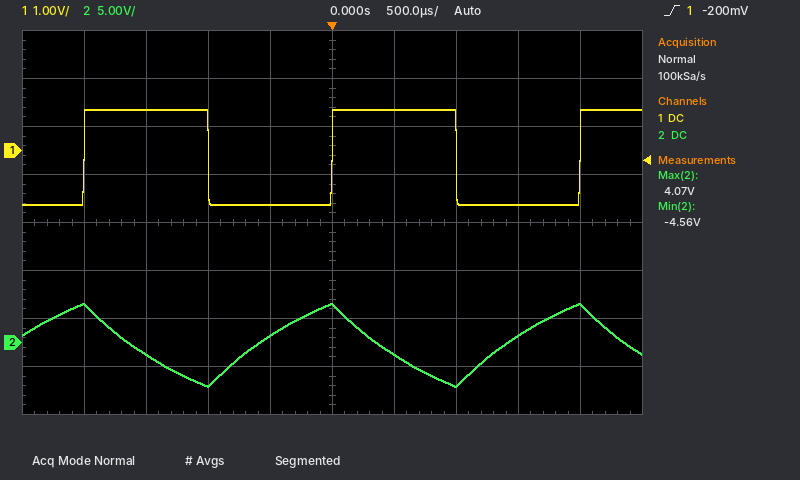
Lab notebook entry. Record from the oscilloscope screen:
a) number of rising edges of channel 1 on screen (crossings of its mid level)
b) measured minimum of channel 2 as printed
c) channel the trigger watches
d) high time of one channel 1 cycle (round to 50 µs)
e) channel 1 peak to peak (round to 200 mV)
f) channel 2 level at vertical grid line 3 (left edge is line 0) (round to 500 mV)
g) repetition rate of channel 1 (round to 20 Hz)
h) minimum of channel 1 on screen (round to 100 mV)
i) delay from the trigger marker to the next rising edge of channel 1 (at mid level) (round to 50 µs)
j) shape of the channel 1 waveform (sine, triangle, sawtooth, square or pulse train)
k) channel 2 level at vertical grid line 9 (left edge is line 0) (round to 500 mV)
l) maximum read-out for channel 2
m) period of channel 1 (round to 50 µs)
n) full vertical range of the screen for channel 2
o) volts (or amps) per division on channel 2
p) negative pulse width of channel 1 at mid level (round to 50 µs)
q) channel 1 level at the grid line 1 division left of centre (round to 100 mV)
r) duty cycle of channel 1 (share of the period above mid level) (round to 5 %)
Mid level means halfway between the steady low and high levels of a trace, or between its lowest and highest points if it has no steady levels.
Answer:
3
-4.56 V
channel 1
1.00 ms
2.0 V
-4.5 V
500 Hz
-1.1 V
2.00 ms
square
4.0 V
4.07 V
2.00 ms
40 V
5 V
1.00 ms
-1.1 V
50 %
